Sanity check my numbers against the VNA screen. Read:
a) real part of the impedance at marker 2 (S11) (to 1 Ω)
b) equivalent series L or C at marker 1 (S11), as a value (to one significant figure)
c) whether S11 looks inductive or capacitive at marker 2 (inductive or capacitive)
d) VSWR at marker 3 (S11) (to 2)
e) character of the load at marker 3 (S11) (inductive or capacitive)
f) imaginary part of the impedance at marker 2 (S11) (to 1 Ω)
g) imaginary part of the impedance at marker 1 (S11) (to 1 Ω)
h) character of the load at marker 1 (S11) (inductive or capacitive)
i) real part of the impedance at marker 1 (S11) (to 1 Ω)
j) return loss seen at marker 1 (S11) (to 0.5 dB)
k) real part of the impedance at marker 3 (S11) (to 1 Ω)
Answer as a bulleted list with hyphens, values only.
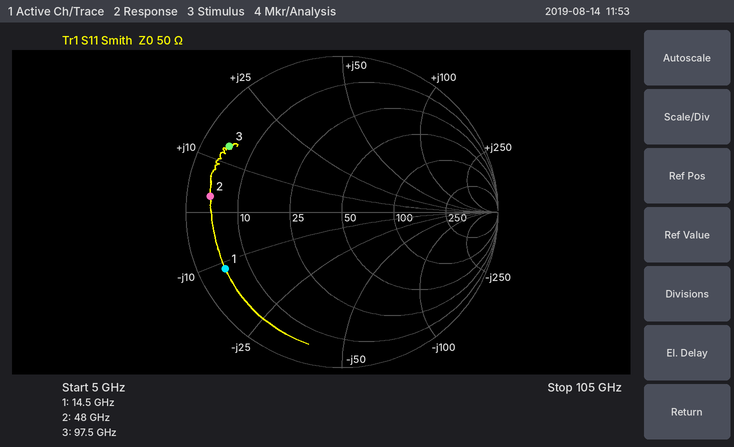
- 4 Ω
- 1.0 pF
- inductive
- 12
- inductive
- +3 Ω
- -11 Ω
- capacitive
- 5 Ω
- 1.5 dB
- 5 Ω
